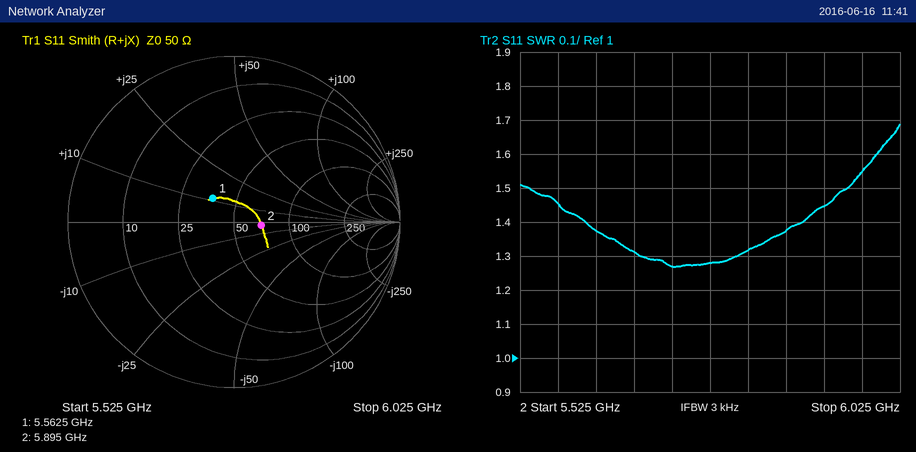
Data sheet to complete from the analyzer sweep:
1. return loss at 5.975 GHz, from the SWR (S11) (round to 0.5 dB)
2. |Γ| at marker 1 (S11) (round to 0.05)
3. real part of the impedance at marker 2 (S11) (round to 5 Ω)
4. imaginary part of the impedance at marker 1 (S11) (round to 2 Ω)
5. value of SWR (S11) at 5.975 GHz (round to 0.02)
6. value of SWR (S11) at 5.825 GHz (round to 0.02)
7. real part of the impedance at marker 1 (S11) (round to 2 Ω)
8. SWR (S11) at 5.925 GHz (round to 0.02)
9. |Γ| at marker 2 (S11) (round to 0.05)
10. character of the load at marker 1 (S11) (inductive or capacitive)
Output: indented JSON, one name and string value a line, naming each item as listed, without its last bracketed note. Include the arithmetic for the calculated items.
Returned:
{
  "return loss at 5.975 GHz, from the SWR (S11)": "−20 log10((1.54 − 1)/(1.54 + 1)) ≈ 13.4 dB, so 13.5 dB to the nearest 0.5 dB",
  "|Γ| at marker 1 (S11)": "0.20",
  "real part of the impedance at marker 2 (S11)": "70 Ω",
  "imaginary part of the impedance at marker 1 (S11)": "+12 Ω",
  "value of SWR (S11) at 5.975 GHz": "1.54",
  "value of SWR (S11) at 5.825 GHz": "1.32",
  "real part of the impedance at marker 1 (S11)": "38 Ω",
  "SWR (S11) at 5.925 GHz": "1.44",
  "|Γ| at marker 2 (S11)": "0.15",
  "character of the load at marker 1 (S11)": "inductive"
}
